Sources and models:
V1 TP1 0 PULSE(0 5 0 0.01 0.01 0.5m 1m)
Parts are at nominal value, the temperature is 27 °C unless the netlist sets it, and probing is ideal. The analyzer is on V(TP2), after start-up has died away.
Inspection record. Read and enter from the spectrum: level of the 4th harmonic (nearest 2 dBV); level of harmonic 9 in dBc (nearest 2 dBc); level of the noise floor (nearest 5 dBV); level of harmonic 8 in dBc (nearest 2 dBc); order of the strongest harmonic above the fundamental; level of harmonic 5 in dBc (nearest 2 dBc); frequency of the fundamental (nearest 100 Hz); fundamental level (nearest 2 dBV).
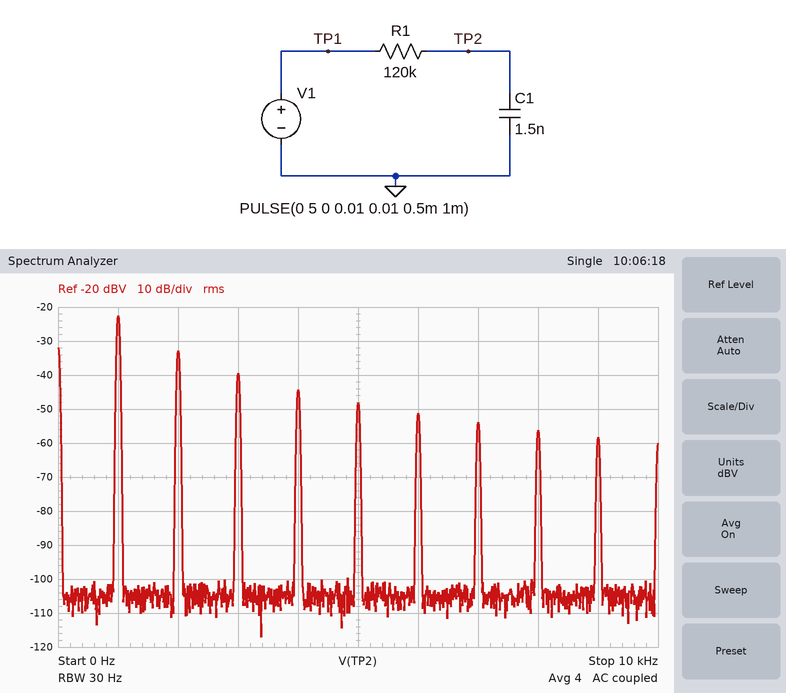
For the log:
-44 dBV
-36 dBc
-105 dBV
-34 dBc
2
-26 dBc
1.0 kHz
-22 dBV
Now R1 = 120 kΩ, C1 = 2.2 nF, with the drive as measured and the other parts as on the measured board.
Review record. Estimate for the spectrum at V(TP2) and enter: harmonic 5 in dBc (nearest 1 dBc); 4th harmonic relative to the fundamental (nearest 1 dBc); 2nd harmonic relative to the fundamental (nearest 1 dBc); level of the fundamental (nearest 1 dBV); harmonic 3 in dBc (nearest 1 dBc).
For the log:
-27 dBc
-23 dBc
-11 dBc
-25 dBV
-18 dBc
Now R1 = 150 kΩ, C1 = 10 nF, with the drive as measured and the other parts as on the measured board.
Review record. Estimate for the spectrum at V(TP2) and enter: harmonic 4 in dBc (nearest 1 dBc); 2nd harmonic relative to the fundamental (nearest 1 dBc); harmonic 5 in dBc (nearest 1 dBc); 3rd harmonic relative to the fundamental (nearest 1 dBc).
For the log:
-24 dBc
-12 dBc
-28 dBc
-19 dBc
